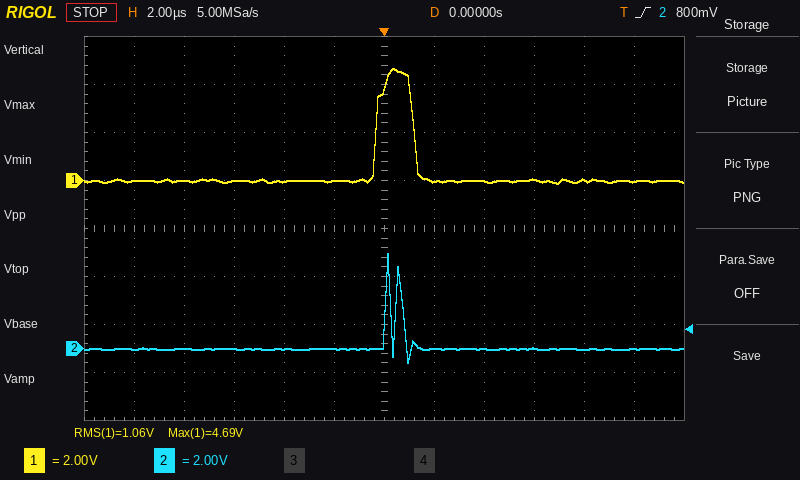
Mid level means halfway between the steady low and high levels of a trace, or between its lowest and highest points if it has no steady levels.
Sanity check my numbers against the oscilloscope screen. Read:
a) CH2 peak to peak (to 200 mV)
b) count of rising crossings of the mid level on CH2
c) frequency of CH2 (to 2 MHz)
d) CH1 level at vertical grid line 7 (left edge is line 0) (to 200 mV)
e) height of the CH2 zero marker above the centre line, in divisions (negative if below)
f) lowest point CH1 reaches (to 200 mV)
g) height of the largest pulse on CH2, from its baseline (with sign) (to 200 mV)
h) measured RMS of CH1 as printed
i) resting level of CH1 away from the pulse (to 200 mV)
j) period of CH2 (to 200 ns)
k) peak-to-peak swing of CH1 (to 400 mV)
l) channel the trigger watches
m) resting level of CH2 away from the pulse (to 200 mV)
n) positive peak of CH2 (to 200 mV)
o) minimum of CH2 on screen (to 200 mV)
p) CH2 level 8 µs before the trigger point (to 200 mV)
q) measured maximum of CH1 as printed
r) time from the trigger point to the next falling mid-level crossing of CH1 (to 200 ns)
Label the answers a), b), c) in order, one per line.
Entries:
a) 4.6 V
b) 2
c) 2 MHz
d) 0.0 V
e) -2.5 div
f) -200 mV
g) +4.0 V
h) 1.06 V
i) 0.0 V
j) 400 ns
k) 4.8 V
l) CH2
m) 0.0 V
n) 4.0 V
o) -600 mV
p) 0.0 V
q) 4.69 V
r) 1.2 µs
